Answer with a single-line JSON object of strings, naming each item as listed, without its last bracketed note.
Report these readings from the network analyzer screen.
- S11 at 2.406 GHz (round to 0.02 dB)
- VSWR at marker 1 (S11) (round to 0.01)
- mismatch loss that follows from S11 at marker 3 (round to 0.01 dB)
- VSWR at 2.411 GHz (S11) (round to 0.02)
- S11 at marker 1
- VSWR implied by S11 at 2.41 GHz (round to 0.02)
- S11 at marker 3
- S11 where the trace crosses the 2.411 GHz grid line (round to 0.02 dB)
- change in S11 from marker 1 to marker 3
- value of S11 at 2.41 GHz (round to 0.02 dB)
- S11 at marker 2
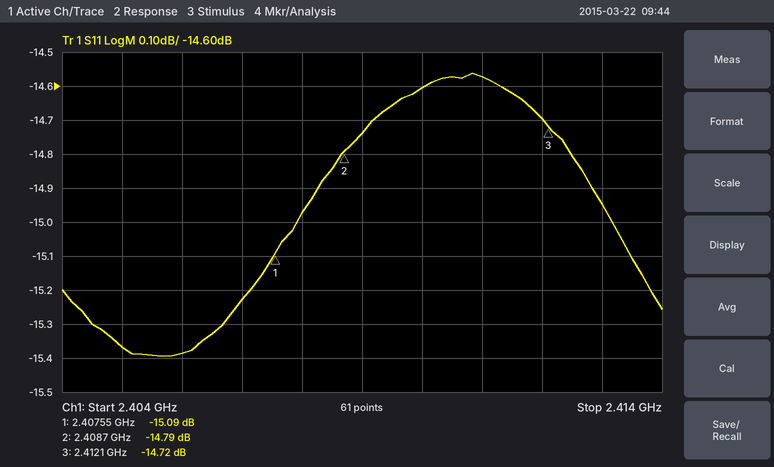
{"S11 at 2.406 GHz": "-15.38 dB", "VSWR at marker 1 (S11)": "1.43", "mismatch loss that follows from S11 at marker 3": "0.15 dB", "VSWR at 2.411 GHz (S11)": "1.46", "S11 at marker 1": "-15.09 dB", "VSWR implied by S11 at 2.41 GHz": "1.46", "S11 at marker 3": "-14.72 dB", "S11 where the trace crosses the 2.411 GHz grid line": "-14.58 dB", "change in S11 from marker 1 to marker 3": "0.37 dB", "value of S11 at 2.41 GHz": "-14.60 dB", "S11 at marker 2": "-14.79 dB"}
